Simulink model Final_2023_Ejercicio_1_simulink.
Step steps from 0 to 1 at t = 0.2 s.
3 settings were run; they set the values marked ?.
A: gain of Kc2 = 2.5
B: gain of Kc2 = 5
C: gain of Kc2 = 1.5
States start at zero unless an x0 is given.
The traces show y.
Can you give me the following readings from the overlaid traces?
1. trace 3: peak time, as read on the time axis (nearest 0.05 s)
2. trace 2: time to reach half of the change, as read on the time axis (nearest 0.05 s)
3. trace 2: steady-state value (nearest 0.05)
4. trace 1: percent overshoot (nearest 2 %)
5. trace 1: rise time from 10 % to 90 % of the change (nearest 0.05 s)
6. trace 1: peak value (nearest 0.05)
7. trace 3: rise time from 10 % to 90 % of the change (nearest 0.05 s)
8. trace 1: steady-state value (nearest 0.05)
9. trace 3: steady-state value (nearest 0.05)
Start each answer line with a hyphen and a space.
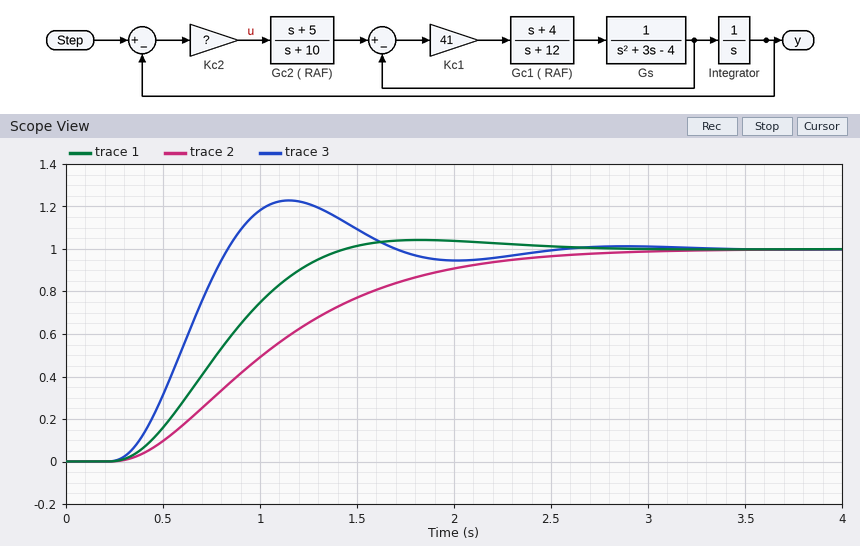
- 1.15 s
- 1.00 s
- 1.00
- 4 %
- 0.75 s
- 1.05
- 0.40 s
- 1.00
- 1.00
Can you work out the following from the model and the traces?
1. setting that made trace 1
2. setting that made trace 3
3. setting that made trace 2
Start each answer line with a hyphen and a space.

- A
- B
- C
